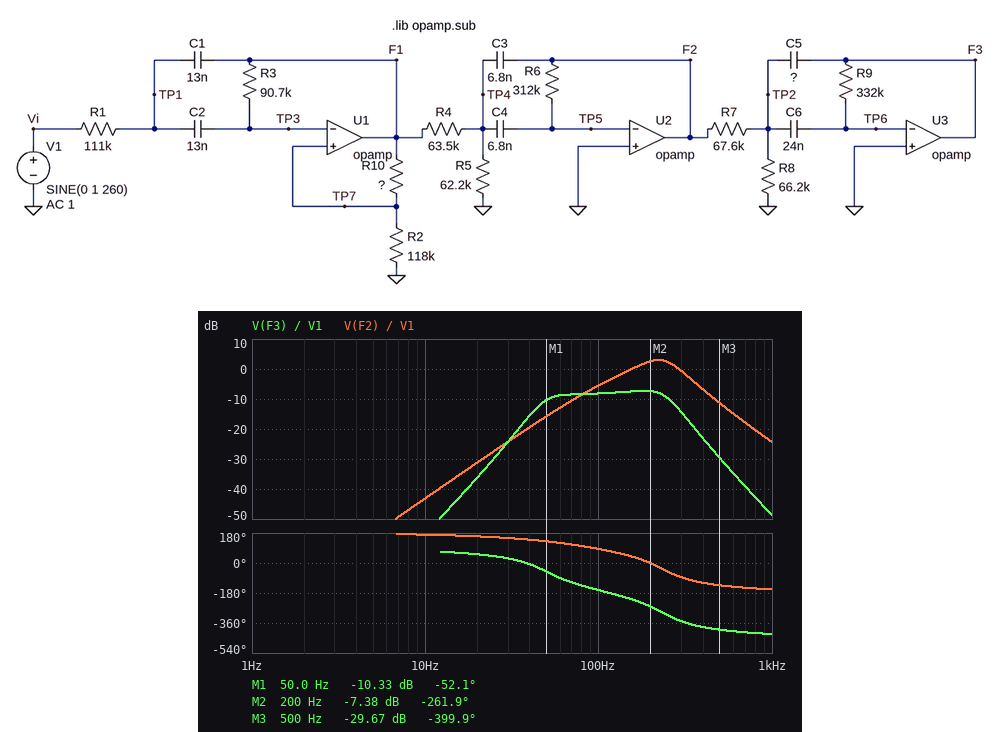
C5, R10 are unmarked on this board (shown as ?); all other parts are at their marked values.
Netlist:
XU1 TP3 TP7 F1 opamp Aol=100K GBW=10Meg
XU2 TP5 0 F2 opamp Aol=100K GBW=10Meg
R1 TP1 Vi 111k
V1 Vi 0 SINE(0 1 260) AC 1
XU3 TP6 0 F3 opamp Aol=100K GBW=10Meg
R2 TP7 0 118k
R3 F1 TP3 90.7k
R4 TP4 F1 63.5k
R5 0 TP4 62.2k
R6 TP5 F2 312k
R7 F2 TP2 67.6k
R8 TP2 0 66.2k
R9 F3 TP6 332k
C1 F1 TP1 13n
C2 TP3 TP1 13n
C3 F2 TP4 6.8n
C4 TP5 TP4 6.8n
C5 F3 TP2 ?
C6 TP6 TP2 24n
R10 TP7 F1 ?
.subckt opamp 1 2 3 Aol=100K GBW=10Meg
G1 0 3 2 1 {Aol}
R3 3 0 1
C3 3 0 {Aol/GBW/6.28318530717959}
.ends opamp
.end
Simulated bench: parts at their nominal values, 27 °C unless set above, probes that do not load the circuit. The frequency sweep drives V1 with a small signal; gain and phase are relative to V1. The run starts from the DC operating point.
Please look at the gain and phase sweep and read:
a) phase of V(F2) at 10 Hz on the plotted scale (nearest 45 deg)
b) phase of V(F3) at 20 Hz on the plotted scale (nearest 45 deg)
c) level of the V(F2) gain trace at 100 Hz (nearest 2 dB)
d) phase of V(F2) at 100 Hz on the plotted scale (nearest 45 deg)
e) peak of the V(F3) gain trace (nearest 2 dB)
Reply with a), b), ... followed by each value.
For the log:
a) 180 deg
b) 45 deg
c) -6 dB
d) 90 deg
e) -8 dB
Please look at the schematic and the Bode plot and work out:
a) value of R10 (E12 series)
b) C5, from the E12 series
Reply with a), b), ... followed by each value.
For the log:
a) 270 kΩ
b) 39 nF
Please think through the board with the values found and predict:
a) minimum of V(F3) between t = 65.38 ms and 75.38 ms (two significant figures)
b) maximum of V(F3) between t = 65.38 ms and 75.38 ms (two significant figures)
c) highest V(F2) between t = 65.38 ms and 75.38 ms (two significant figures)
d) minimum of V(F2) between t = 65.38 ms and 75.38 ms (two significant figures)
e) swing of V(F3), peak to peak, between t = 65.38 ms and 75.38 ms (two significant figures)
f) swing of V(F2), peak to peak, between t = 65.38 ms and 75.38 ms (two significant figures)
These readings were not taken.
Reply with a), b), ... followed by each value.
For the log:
a) -300 mV
b) 300 mV
c) 1.2 V
d) -1.2 V
e) 590 mV
f) 2.5 V
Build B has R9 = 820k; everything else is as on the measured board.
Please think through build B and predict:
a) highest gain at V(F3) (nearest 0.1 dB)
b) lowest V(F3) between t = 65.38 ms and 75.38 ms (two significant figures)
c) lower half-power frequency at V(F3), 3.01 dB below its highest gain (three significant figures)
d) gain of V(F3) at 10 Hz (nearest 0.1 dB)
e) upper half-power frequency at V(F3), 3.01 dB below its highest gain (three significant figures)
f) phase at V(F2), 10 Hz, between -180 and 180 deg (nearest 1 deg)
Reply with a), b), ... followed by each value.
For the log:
a) -7.5 dB
b) -290 mV
c) 30.8 Hz
d) -46.5 dB
e) 258 Hz
f) 170 deg
